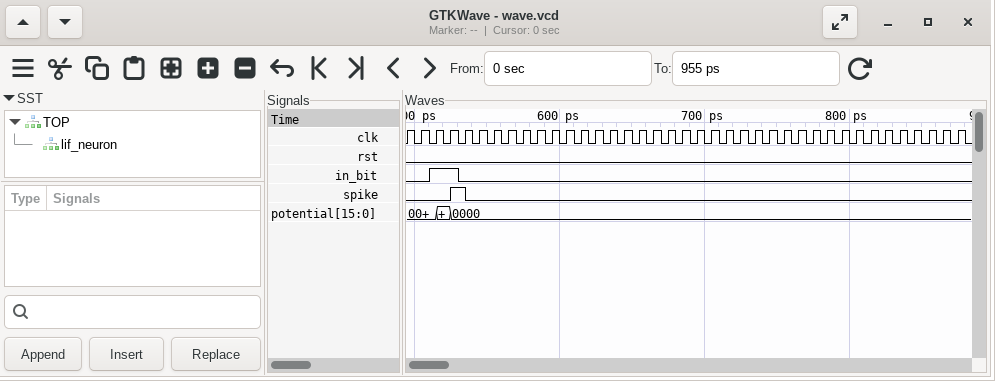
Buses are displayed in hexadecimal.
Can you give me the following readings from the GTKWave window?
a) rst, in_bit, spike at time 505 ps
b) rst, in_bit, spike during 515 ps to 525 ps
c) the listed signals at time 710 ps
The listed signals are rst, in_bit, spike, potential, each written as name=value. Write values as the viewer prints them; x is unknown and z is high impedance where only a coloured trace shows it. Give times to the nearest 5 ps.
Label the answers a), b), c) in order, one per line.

a) rst=0, in_bit=0, spike=0
b) rst=0, in_bit=1, spike=0
c) rst=0, in_bit=0, spike=0, potential=0000
